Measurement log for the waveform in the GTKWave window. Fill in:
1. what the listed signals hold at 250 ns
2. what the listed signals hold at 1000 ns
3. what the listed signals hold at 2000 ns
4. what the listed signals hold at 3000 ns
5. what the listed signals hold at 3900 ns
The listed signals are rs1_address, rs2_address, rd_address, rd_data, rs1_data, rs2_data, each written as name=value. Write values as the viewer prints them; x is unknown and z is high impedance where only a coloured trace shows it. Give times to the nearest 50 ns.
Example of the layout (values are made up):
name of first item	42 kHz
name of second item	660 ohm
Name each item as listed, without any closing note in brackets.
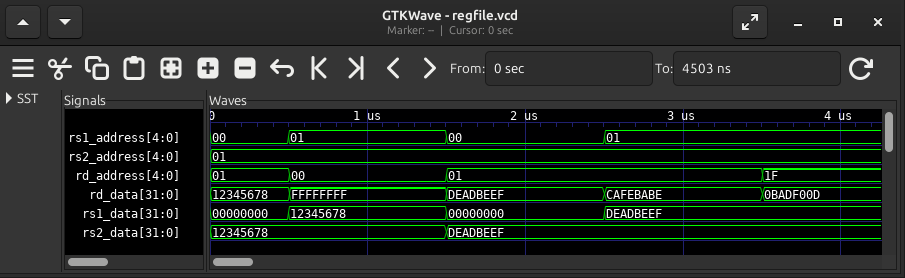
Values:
what the listed signals hold at 250 ns	rs1_address=00, rs2_address=01, rd_address=01, rd_data=12345678, rs1_data=00000000, rs2_data=12345678
what the listed signals hold at 1000 ns	rs1_address=01, rs2_address=01, rd_address=00, rd_data=FFFFFFFF, rs1_data=12345678, rs2_data=12345678
what the listed signals hold at 2000 ns	rs1_address=00, rs2_address=01, rd_address=01, rd_data=DEADBEEF, rs1_data=00000000, rs2_data=DEADBEEF
what the listed signals hold at 3000 ns	rs1_address=01, rs2_address=01, rd_address=01, rd_data=CAFEBABE, rs1_data=DEADBEEF, rs2_data=DEADBEEF
what the listed signals hold at 3900 ns	rs1_address=01, rs2_address=01, rd_address=1F, rd_data=0BADF00D, rs1_data=DEADBEEF, rs2_data=DEADBEEF
